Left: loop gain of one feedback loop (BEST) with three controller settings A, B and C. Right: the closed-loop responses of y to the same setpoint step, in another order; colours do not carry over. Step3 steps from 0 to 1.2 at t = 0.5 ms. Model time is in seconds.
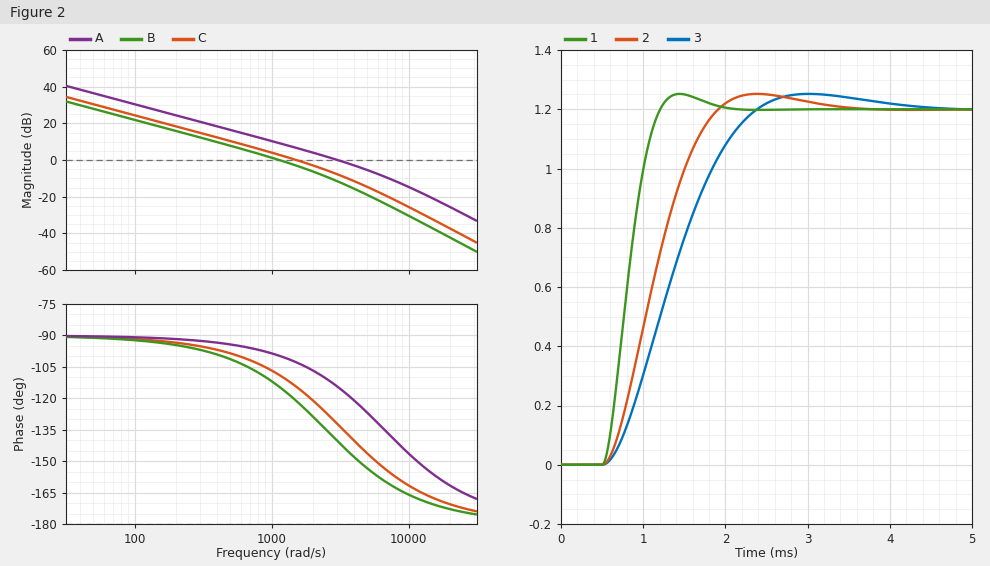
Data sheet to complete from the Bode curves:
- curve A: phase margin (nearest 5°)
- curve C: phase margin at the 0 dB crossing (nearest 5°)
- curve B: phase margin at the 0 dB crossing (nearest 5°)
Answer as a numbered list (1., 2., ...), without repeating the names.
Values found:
1. 65°
2. 65°
3. 65°
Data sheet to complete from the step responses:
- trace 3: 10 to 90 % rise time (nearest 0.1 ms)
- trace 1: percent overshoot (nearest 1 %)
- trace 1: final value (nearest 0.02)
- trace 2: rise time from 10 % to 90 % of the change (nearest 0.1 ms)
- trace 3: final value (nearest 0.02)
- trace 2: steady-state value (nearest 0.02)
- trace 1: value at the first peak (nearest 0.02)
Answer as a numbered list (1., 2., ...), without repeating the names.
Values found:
1. 1.2 ms
2. 4 %
3. 1.20
4. 0.9 ms
5. 1.20
6. 1.20
7. 1.26
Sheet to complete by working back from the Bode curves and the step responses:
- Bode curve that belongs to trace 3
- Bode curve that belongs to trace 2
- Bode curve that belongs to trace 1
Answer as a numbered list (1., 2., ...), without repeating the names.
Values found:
1. B
2. C
3. A
